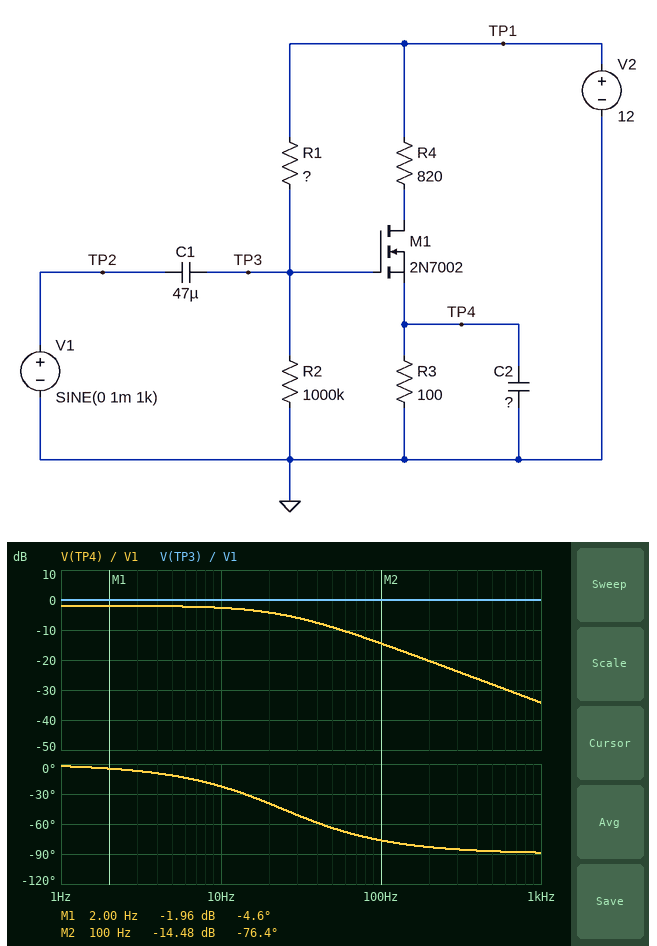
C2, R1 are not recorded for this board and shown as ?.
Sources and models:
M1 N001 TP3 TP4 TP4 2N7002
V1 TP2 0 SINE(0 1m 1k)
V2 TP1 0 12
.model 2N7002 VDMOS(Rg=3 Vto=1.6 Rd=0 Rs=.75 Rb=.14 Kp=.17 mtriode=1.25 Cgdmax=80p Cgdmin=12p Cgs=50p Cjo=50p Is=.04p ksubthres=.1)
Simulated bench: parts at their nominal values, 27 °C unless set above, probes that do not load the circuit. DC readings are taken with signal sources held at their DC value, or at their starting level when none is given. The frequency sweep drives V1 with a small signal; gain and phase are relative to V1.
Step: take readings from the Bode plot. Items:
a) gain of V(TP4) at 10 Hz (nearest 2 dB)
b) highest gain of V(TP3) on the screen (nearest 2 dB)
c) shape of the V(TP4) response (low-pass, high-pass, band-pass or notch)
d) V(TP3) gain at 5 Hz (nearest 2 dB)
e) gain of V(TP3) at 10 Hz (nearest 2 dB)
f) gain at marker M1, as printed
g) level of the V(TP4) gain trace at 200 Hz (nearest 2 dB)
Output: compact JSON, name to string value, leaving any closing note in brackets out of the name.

{"gain of V(TP4) at 10 Hz": "-2 dB", "highest gain of V(TP3) on the screen": "0 dB", "shape of the V(TP4) response": "low-pass", "V(TP3) gain at 5 Hz": "0 dB", "gain of V(TP3) at 10 Hz": "0 dB", "gain at marker M1, as printed": "-1.96 dB", "level of the V(TP4) gain trace at 200 Hz": "-20 dB"}
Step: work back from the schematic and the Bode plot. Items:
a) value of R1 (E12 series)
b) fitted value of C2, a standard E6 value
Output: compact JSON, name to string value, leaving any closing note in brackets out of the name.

{"value of R1": "3.9 MΩ", "fitted value of C2, a standard E6 value": "330 µF"}
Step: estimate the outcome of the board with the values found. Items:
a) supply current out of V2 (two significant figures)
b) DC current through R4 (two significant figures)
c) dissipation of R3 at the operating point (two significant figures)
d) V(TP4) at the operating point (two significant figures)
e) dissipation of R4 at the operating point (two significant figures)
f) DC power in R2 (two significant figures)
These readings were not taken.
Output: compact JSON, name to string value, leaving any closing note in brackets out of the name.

{"supply current out of V2": "5.9 mA", "DC current through R4": "5.9 mA", "dissipation of R3 at the operating point": "3.5 mW", "V(TP4) at the operating point": "590 mV", "dissipation of R4 at the operating point": "28 mW", "DC power in R2": "6.0 µW"}
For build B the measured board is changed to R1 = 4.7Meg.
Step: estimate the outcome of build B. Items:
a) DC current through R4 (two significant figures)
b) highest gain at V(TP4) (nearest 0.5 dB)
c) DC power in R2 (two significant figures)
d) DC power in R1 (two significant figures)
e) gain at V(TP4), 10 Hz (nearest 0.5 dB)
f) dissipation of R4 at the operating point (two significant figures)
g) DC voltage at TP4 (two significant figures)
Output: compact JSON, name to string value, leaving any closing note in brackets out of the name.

{"DC current through R4": "3.2 mA", "highest gain at V(TP4)": "-2.5 dB", "DC power in R2": "4.4 µW", "DC power in R1": "21 µW", "gain at V(TP4), 10 Hz": "-4.0 dB", "dissipation of R4 at the operating point": "8.6 mW", "DC voltage at TP4": "320 mV"}
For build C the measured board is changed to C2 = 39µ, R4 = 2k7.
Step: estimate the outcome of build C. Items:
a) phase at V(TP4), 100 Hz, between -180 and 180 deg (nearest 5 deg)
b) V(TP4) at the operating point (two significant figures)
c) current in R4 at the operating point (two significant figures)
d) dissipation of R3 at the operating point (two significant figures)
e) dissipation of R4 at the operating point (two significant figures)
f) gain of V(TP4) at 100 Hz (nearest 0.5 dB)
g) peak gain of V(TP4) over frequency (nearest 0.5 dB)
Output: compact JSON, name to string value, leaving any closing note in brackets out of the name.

{"phase at V(TP4), 100 Hz, between -180 and 180 deg": "-65 deg", "V(TP4) at the operating point": "430 mV", "current in R4 at the operating point": "4.3 mA", "dissipation of R3 at the operating point": "1.8 mW", "dissipation of R4 at the operating point": "49 mW", "gain of V(TP4) at 100 Hz": "-54.0 dB", "peak gain of V(TP4) over frequency": "-46.0 dB"}
